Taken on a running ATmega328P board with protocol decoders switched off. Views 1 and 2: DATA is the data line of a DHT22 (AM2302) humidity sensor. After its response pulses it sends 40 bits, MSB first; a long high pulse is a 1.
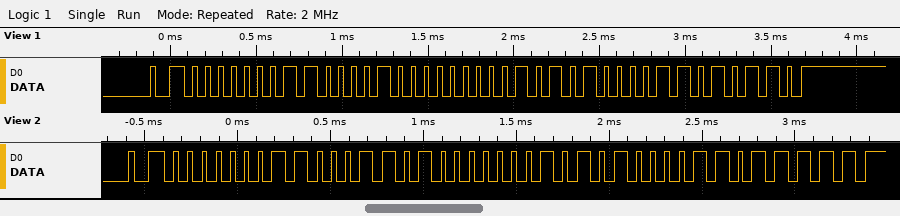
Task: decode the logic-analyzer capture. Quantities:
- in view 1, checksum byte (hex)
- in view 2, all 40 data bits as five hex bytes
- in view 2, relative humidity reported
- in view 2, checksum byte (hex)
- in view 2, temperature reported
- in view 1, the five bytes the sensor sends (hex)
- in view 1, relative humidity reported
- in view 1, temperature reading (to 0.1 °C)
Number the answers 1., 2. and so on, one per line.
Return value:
1. 0xD6
2. 01 8D 01 50 DF
3. 39.7 %
4. 0xDF
5. 33.6 °C
6. 01 84 01 50 D6
7. 38.8 %
8. 33.6 °C
